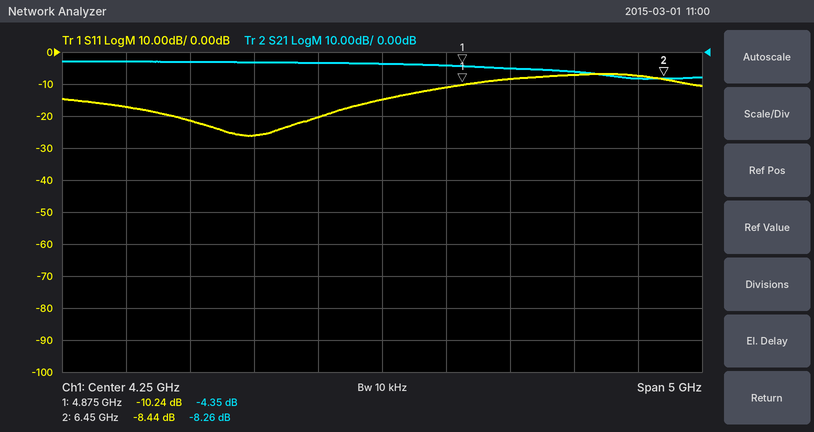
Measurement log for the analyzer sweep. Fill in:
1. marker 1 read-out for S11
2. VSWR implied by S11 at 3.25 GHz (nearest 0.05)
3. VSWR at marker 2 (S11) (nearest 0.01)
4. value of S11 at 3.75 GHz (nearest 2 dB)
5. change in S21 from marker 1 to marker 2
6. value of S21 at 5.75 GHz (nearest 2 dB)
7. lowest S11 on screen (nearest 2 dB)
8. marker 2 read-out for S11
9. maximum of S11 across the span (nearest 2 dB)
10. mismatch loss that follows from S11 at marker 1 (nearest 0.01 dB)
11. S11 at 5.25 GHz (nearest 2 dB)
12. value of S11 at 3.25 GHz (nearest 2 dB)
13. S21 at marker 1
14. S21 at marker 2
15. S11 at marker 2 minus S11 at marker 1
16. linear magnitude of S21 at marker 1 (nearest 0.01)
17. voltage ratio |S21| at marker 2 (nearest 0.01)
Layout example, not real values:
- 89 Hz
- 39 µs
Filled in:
- -10.24 dB
- 1.10
- 2.22
- -20 dB
- -3.91 dB
- -6 dB
- -26 dB
- -8.44 dB
- -6 dB
- 0.43 dB
- -8 dB
- -26 dB
- -4.35 dB
- -8.26 dB
- 1.80 dB
- 0.61
- 0.39
